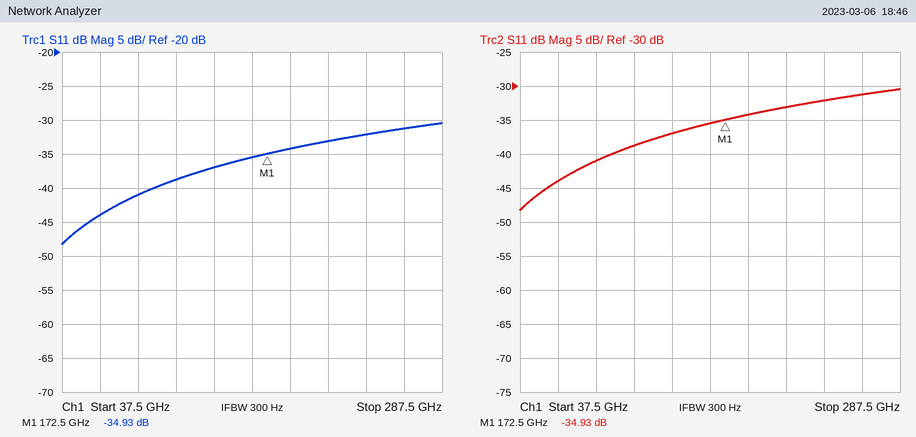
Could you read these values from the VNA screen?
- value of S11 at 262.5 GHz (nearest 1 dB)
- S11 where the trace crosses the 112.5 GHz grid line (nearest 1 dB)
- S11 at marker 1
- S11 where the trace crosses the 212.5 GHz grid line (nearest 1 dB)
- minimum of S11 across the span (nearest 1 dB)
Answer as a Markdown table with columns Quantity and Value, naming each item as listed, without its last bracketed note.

| Quantity | Value |
|---|---|
| value of S11 at 262.5 GHz | -31 dB |
| S11 where the trace crosses the 112.5 GHz grid line | -39 dB |
| S11 at marker 1 | -34.93 dB |
| S11 where the trace crosses the 212.5 GHz grid line | -33 dB |
| minimum of S11 across the span | -48 dB |
